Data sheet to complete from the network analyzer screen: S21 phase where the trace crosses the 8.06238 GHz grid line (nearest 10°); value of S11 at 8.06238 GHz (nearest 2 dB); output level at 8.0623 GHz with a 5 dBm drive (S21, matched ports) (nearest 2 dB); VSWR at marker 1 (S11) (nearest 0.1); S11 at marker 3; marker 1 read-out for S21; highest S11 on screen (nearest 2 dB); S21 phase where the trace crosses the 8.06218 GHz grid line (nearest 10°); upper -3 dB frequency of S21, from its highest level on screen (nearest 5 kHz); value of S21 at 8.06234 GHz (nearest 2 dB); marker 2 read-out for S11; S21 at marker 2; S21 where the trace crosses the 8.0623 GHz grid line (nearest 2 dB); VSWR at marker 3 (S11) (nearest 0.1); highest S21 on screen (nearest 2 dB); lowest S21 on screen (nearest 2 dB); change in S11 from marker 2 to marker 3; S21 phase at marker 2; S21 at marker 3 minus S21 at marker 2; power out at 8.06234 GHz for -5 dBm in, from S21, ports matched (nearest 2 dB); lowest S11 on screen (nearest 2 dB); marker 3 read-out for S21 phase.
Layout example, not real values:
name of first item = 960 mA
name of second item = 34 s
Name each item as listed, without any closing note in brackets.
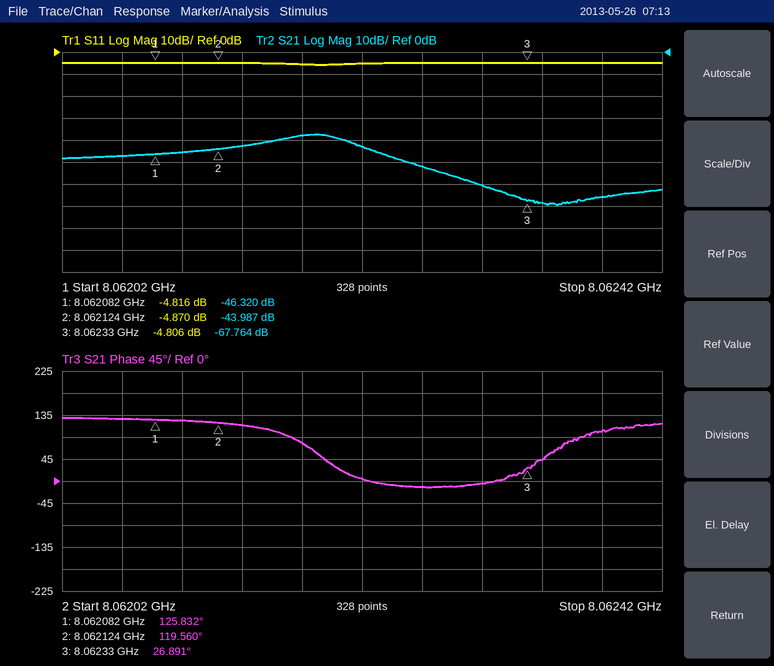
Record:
S21 phase where the trace crosses the 8.06238 GHz grid line = 100°
value of S11 at 8.06238 GHz = -4 dB
output level at 8.0623 GHz with a 5 dBm drive (S21, matched ports) = -56 dBm
VSWR at marker 1 (S11) = 3.7
S11 at marker 3 = -4.806 dB
marker 1 read-out for S21 = -46.320 dB
highest S11 on screen = -4 dB
S21 phase where the trace crosses the 8.06218 GHz grid line = 80°
upper -3 dB frequency of S21, from its highest level on screen = 8.062210 GHz
value of S21 at 8.06234 GHz = -68 dB
marker 2 read-out for S11 = -4.870 dB
S21 at marker 2 = -43.987 dB
S21 where the trace crosses the 8.0623 GHz grid line = -60 dB
VSWR at marker 3 (S11) = 3.7
highest S21 on screen = -38 dB
lowest S21 on screen = -70 dB
change in S11 from marker 2 to marker 3 = 0.064 dB
S21 phase at marker 2 = 119.560°
S21 at marker 3 minus S21 at marker 2 = -23.777 dB
power out at 8.06234 GHz for -5 dBm in, from S21, ports matched = -74 dBm
lowest S11 on screen = -6 dB
marker 3 read-out for S21 phase = 26.891°
